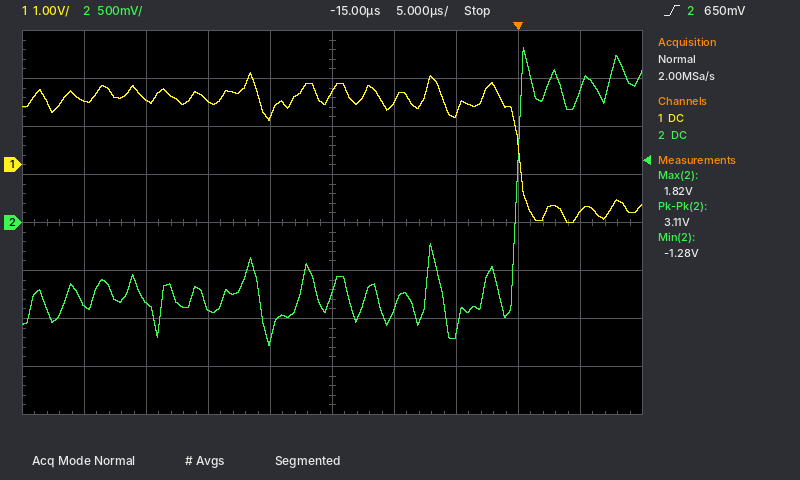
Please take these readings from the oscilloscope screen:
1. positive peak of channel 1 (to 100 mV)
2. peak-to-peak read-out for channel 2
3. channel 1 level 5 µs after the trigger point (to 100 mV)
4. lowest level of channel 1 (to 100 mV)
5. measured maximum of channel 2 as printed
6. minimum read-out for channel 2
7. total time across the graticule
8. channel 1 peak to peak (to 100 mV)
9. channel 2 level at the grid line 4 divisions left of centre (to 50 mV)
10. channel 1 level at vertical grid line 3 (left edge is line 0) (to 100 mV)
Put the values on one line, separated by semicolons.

1.9 V; 3.11 V; -1.0 V; -1.2 V; 1.82 V; -1.28 V; 50 µs; 3.1 V; -850 mV; 1.3 V
